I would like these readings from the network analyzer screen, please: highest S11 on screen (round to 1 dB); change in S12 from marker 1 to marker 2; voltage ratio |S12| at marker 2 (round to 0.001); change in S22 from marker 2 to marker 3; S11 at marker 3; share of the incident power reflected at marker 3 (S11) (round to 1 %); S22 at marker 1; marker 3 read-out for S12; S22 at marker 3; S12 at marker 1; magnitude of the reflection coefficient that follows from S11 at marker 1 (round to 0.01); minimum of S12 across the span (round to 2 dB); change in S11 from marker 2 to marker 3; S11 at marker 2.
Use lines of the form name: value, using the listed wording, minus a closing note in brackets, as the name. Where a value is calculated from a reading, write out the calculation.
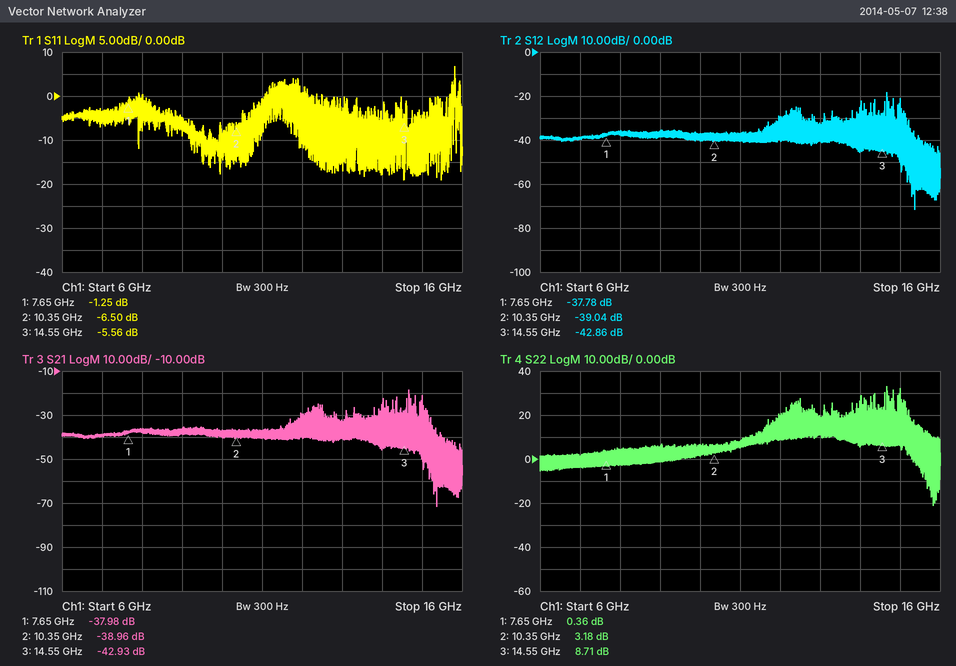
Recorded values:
highest S11 on screen: 7 dB
change in S12 from marker 1 to marker 2: -39.04 − (-37.78) = -1.26 dB
voltage ratio |S12| at marker 2: 10^(-39.04/20) ≈ 0.011
change in S22 from marker 2 to marker 3: 8.71 − (3.18) = 5.53 dB
S11 at marker 3: -5.56 dB
share of the incident power reflected at marker 3 (S11): 10^(-5.56/10) ≈ 28 %
S22 at marker 1: 0.36 dB
marker 3 read-out for S12: -42.86 dB
S22 at marker 3: 8.71 dB
S12 at marker 1: -37.78 dB
magnitude of the reflection coefficient that follows from S11 at marker 1: 10^(-1.25/20) ≈ 0.87
minimum of S12 across the span: -72 dB
change in S11 from marker 2 to marker 3: -5.56 − (-6.5) = 0.94 dB
S11 at marker 2: -6.50 dB
